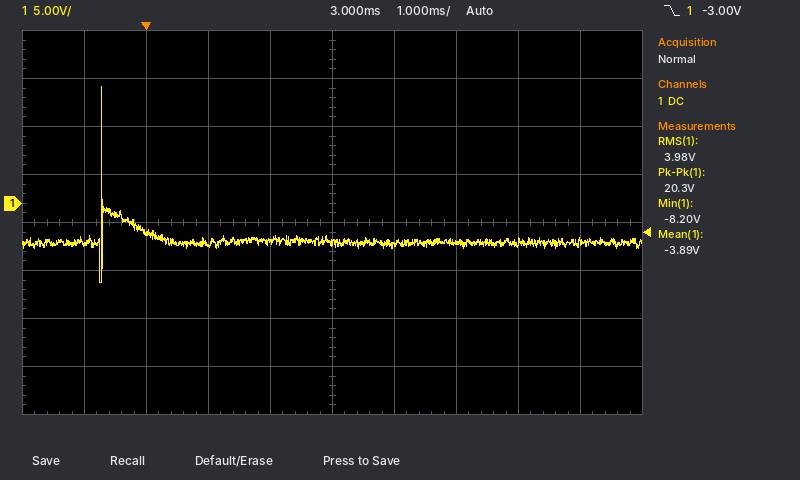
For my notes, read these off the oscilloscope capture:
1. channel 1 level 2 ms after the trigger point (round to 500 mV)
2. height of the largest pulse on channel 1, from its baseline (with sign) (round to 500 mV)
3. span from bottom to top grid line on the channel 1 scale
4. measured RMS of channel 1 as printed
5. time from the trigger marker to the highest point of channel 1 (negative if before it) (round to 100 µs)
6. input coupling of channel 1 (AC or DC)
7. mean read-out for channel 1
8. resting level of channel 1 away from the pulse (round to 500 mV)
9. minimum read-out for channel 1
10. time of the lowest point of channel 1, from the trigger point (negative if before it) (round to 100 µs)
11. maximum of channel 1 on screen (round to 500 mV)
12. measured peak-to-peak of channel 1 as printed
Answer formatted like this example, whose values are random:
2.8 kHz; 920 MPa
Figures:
-4.0 V; +16.0 V; 40 V; 3.98 V; -700 µs; DC; -3.89 V; -4.0 V; -8.20 V; -700 µs; 12.0 V; 20.3 V
